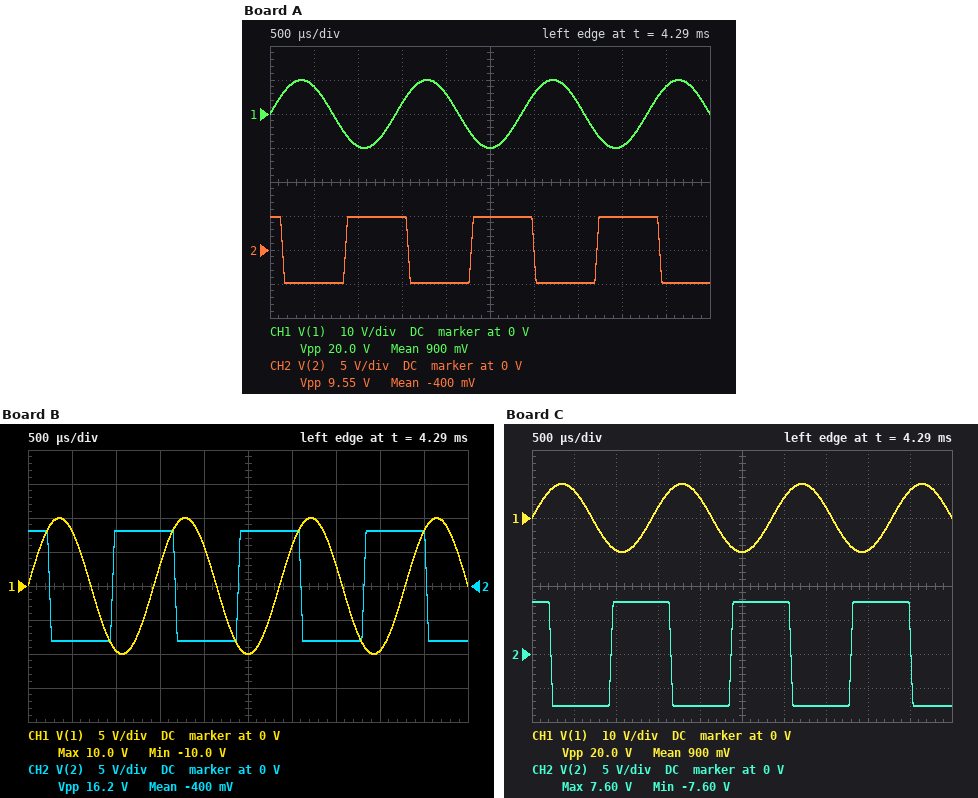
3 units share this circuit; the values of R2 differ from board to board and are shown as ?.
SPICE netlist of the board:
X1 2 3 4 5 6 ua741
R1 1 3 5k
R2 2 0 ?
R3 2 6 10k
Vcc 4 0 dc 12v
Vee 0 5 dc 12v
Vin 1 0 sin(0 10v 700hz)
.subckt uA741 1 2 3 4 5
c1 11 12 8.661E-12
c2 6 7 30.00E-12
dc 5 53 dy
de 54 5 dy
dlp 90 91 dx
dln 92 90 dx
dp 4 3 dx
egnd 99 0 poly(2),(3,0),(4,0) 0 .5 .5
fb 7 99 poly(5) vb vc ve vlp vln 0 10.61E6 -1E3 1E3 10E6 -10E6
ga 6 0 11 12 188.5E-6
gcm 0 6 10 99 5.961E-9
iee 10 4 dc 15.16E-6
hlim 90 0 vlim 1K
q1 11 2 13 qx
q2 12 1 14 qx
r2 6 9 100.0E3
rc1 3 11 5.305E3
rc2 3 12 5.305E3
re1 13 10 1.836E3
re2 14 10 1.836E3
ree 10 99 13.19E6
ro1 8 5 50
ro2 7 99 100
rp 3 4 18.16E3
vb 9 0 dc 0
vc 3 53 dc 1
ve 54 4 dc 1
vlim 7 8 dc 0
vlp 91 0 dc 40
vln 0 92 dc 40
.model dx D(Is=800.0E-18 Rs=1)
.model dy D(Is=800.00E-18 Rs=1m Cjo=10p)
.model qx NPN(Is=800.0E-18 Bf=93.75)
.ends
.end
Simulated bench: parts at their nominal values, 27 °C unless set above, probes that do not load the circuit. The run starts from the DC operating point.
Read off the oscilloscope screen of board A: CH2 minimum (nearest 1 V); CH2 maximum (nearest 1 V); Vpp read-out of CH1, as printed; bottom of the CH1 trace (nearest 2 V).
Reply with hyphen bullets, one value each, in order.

- -5 V
- 5 V
- 20.0 V
- -10 V
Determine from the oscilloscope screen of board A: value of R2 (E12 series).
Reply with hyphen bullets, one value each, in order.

- 6.8 kΩ
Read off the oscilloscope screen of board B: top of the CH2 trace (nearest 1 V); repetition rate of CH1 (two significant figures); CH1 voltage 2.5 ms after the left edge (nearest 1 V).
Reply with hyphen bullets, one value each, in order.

- 8 V
- 700 Hz
- -10 V
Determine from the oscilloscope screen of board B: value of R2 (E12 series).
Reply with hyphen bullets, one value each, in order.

- 22 kΩ
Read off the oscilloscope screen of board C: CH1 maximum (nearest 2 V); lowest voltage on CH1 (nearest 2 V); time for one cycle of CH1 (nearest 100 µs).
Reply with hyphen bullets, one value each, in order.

- 10 V
- -10 V
- 1.4 ms
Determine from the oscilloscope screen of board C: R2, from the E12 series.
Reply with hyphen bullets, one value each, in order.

- 18 kΩ
